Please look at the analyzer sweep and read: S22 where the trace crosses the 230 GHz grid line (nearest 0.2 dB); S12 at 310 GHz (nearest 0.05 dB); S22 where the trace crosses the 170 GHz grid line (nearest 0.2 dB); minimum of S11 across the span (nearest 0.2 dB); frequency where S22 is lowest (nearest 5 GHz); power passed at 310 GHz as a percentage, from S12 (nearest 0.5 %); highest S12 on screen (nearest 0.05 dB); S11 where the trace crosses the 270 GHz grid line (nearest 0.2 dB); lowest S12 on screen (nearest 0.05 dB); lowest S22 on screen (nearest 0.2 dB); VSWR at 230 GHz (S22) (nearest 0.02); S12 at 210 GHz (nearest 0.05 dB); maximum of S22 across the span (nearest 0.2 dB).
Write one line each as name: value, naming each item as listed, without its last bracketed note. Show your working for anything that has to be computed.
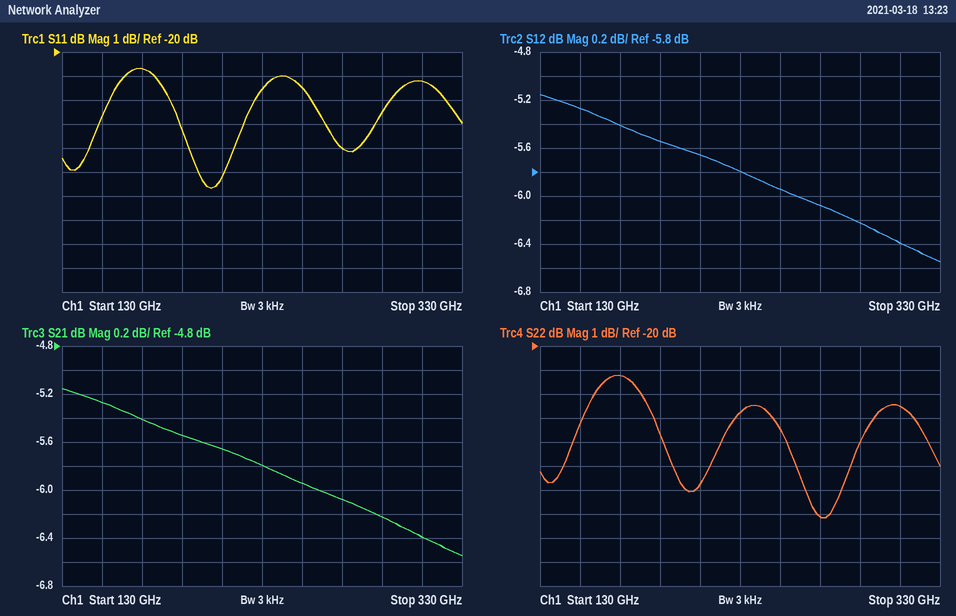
S22 where the trace crosses the 230 GHz grid line: -22.8 dB
S12 at 310 GHz: -6.40 dB
S22 where the trace crosses the 170 GHz grid line: -21.2 dB
minimum of S11 across the span: -25.6 dB
frequency where S22 is lowest: 270 GHz
power passed at 310 GHz as a percentage, from S12: 10^(-6.4/10) ≈ 22.9 %, so 23.0 % to the nearest 0.5 %
highest S12 on screen: -5.15 dB
S11 where the trace crosses the 270 GHz grid line: -24.0 dB
lowest S12 on screen: -6.55 dB
lowest S22 on screen: -27.2 dB
VSWR at 230 GHz (S22): |Γ| = 10^(-22.8/20) = 0.0724; VSWR = (1 + 0.0724)/(1 − 0.0724) ≈ 1.16
S12 at 210 GHz: -5.65 dB
maximum of S22 across the span: -21.2 dB
